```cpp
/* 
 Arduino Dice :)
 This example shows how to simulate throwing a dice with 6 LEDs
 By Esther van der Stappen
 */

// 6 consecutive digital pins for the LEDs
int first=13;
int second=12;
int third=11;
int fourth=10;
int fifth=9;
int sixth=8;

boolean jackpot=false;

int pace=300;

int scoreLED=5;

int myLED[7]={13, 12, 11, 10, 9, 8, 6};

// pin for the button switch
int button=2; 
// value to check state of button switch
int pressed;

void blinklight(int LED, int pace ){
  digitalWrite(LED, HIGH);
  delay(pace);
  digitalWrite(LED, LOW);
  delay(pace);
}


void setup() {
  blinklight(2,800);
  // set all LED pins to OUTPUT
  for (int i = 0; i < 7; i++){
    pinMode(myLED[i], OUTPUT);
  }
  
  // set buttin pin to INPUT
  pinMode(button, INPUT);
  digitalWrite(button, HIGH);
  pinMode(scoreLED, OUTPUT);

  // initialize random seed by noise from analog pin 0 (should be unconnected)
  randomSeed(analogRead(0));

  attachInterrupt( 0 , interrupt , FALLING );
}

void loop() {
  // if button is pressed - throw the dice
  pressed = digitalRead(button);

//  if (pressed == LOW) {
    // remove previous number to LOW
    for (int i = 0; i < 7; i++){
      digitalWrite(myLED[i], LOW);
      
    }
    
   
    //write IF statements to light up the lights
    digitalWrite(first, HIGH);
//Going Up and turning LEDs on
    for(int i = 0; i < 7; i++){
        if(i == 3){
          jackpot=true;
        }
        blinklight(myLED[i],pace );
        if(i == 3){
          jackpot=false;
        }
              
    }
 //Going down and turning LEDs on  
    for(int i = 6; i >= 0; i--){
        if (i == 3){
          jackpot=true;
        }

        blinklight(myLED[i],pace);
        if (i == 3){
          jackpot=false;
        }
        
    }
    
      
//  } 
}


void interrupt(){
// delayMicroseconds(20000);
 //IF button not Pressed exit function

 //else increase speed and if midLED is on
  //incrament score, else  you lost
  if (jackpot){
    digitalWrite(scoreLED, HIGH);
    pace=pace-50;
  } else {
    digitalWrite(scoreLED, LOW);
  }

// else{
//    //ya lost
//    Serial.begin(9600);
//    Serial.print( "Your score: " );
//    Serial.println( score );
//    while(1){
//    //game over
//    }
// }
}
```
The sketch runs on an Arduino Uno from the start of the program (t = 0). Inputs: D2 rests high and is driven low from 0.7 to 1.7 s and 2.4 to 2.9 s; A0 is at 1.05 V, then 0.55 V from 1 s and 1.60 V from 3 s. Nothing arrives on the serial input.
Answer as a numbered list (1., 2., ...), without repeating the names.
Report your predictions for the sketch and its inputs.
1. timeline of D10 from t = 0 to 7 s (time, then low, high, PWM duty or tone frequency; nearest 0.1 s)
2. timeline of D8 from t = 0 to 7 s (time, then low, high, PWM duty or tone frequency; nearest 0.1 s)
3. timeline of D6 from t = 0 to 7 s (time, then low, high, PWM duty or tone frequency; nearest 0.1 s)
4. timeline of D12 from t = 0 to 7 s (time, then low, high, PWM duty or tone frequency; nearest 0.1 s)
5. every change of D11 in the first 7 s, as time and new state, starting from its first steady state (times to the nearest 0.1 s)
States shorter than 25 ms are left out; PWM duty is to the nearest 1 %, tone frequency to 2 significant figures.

1. 1.6 s low; 3.4 s high; 3.7 s low
2. 1.6 s low; 4.6 s high; 4.9 s low; 6.4 s high; 6.7 s low
3. 1.6 s low; 5.2 s high; 5.5 s low; 5.8 s high; 6.1 s low
4. 1.6 s low; 2.2 s high; 2.5 s low
5. 1.6 s low; 2.8 s high; 3.1 s low
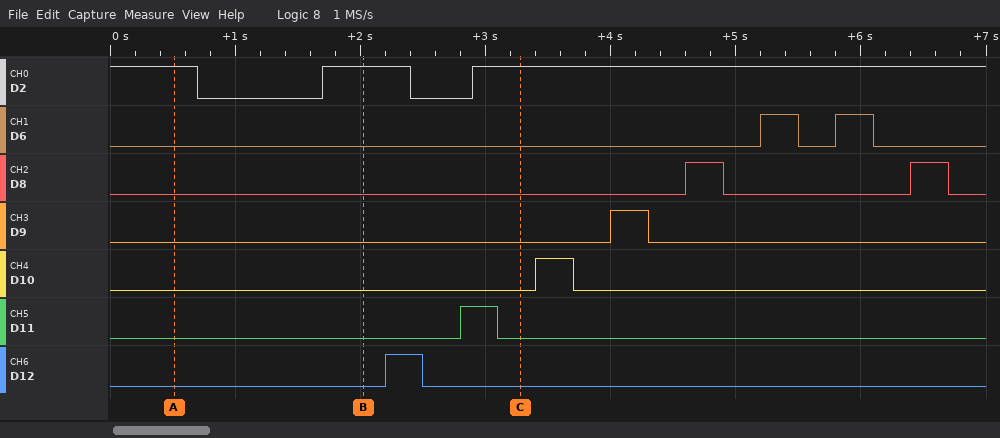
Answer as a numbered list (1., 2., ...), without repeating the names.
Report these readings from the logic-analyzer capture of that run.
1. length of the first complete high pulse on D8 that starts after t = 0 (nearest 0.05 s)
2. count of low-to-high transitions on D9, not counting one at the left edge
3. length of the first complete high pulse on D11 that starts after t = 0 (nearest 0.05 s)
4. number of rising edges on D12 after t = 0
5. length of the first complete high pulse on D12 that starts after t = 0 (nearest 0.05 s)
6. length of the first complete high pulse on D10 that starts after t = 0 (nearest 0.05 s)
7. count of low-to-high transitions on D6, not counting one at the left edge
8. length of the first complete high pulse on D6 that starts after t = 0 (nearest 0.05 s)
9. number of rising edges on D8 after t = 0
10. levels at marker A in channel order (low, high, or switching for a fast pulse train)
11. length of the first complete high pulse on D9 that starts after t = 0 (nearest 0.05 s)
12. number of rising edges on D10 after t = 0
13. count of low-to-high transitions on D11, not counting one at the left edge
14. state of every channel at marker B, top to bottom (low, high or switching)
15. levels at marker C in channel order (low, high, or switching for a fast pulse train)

1. 0.30 s
2. 1
3. 0.30 s
4. 1
5. 0.30 s
6. 0.30 s
7. 2
8. 0.30 s
9. 2
10. D2 high, D6 low, D8 low, D9 low, D10 low, D11 low, D12 low
11. 0.30 s
12. 1
13. 1
14. D2 high, D6 low, D8 low, D9 low, D10 low, D11 low, D12 low
15. D2 high, D6 low, D8 low, D9 low, D10 low, D11 low, D12 low
